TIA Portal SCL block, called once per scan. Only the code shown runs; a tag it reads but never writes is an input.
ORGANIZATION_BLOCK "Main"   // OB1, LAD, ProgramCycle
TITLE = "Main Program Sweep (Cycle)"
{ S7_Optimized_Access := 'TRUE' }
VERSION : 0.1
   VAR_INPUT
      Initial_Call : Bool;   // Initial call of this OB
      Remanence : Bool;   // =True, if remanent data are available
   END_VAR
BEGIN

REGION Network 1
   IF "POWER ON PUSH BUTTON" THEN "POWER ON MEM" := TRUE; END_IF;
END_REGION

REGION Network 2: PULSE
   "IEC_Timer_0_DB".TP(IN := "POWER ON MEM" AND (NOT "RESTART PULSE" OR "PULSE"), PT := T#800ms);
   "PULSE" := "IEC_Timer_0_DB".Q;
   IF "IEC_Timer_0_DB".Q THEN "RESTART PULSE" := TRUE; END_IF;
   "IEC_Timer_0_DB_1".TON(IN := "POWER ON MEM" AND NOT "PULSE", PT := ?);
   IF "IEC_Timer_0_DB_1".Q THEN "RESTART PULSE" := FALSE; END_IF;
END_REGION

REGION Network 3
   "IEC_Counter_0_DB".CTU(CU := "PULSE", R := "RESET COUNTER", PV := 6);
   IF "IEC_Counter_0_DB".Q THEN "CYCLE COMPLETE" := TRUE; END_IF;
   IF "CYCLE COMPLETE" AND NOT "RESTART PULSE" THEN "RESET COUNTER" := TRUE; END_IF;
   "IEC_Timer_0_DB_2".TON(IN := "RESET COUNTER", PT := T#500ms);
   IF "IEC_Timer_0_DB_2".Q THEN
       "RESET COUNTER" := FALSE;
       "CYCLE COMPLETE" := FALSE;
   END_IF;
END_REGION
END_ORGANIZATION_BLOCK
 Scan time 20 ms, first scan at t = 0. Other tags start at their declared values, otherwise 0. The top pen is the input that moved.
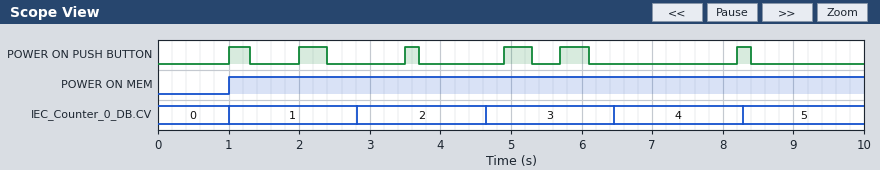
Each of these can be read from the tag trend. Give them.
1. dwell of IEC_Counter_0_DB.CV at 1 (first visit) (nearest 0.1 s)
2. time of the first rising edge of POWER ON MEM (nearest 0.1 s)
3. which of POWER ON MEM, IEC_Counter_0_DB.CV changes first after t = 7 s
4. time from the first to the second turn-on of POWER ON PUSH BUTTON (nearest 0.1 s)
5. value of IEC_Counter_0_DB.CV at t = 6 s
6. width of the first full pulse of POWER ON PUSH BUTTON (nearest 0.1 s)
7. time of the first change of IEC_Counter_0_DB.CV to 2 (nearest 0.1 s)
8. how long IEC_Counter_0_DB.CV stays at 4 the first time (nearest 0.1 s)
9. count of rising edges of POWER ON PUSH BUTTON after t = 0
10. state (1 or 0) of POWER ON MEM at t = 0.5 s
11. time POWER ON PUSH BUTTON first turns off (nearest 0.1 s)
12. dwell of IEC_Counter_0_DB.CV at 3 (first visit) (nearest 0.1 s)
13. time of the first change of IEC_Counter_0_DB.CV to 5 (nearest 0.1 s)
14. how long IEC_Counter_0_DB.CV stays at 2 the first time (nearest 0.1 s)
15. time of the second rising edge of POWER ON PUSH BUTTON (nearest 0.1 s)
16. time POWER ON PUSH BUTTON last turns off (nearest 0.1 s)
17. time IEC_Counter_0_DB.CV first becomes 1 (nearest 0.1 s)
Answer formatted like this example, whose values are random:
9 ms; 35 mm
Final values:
1.8 s; 1.0 s; IEC_Counter_0_DB.CV; 1.0 s; 3; 0.3 s; 2.8 s; 1.8 s; 6; 0; 1.3 s; 1.8 s; 8.3 s; 1.8 s; 2.0 s; 8.4 s; 1.0 s
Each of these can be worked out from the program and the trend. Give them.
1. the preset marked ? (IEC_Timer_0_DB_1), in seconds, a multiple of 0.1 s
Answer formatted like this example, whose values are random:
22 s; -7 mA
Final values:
1.0 s
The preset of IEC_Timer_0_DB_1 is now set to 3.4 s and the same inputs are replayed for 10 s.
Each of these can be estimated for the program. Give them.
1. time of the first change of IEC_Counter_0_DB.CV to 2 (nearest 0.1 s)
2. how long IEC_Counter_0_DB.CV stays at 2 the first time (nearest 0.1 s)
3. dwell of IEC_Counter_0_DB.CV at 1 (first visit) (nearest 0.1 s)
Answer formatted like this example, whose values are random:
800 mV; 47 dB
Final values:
5.2 s; 4.2 s; 4.2 s
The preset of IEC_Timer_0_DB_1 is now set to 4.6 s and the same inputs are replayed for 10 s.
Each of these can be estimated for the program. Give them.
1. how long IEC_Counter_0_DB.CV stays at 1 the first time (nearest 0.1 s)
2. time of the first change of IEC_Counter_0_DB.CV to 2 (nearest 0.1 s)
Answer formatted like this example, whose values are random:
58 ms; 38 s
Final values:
5.4 s; 6.4 s
